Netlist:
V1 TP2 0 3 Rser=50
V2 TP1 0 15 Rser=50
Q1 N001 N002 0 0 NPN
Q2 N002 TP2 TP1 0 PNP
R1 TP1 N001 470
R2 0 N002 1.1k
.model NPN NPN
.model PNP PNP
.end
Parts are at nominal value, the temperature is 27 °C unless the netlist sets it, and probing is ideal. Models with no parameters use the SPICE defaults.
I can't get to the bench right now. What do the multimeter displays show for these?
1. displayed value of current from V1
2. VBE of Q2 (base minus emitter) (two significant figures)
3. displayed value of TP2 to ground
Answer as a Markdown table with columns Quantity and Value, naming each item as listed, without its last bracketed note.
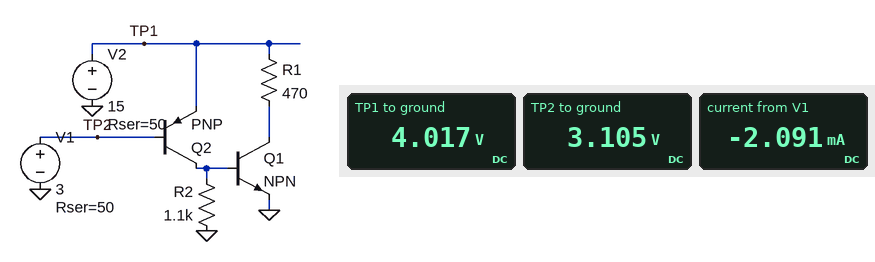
| Quantity | Value |
|---|---|
| displayed value of current from V1 | -2.091 mA |
| VBE of Q2 (base minus emitter) | -910 mV |
| displayed value of TP2 to ground | 3.105 V |
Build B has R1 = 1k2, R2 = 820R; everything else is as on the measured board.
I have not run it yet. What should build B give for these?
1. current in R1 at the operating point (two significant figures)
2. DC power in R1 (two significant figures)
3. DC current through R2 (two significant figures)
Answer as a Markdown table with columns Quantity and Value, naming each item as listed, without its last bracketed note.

| Quantity | Value |
|---|---|
| current in R1 at the operating point | 3.3 mA |
| DC power in R1 | 13 mW |
| DC current through R2 | 1.1 mA |
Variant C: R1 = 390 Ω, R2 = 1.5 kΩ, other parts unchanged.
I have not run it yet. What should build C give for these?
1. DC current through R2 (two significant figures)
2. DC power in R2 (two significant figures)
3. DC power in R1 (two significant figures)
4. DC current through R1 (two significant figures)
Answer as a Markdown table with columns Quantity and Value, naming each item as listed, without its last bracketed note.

| Quantity | Value |
|---|---|
| DC current through R2 | 620 µA |
| DC power in R2 | 580 µW |
| DC power in R1 | 41 mW |
| DC current through R1 | 10 mA |
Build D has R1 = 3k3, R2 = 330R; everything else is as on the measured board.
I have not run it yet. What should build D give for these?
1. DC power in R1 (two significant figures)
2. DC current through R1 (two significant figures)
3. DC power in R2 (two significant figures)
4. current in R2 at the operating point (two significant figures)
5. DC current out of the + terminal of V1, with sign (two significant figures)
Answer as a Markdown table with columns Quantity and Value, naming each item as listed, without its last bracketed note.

| Quantity | Value |
|---|---|
| DC power in R1 | 4.9 mW |
| DC current through R1 | 1.2 mA |
| DC power in R2 | 2.6 mW |
| current in R2 at the operating point | 2.8 mA |
| DC current out of the + terminal of V1, with sign | -2.2 mA |
